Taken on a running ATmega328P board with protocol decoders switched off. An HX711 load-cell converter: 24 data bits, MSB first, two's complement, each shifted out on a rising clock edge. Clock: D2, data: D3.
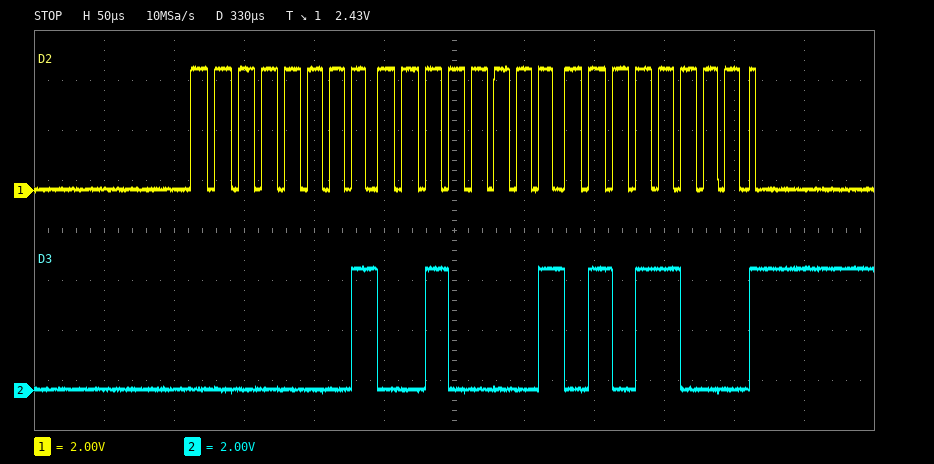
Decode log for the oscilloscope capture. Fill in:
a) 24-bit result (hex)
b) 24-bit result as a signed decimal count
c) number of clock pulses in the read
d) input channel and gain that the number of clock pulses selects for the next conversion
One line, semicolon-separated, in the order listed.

0x012158; 74072; 25; channel A, gain 128
